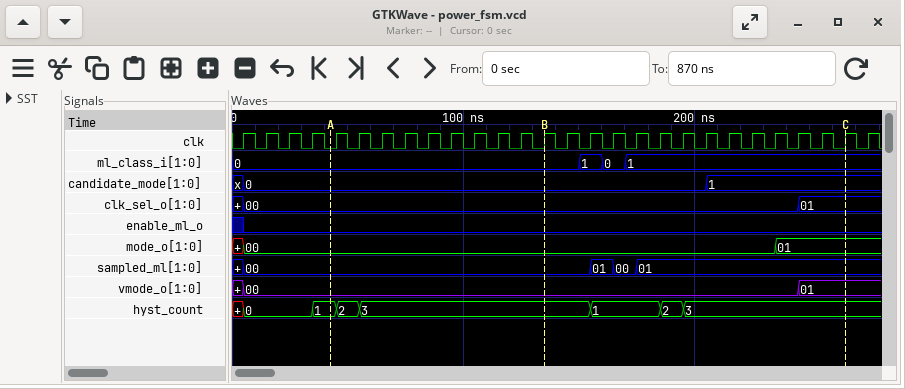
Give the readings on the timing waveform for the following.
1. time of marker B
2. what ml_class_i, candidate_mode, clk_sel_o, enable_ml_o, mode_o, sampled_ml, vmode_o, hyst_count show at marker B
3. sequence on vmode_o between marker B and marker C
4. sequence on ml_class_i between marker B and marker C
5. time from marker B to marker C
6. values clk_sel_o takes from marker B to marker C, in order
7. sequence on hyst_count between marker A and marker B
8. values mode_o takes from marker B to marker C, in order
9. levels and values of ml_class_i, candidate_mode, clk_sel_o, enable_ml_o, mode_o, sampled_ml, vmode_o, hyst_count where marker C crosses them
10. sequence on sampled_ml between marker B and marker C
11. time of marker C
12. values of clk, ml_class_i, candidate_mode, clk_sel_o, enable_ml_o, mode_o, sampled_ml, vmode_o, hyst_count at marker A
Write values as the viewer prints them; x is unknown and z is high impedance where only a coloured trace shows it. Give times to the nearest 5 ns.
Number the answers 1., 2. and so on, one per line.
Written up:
1. 135 ns
2. ml_class_i=0, candidate_mode=0, clk_sel_o=00, enable_ml_o=0, mode_o=00, sampled_ml=00, vmode_o=00, hyst_count=3
3. 00, 01
4. 0, 1, 0, 1
5. 130 ns
6. 00, 01
7. 1, 2, 3
8. 00, 01
9. ml_class_i=1, candidate_mode=1, clk_sel_o=01, enable_ml_o=0, mode_o=01, sampled_ml=01, vmode_o=01, hyst_count=3
10. 00, 01, 00, 01
11. 265 ns
12. clk=0, ml_class_i=0, candidate_mode=0, clk_sel_o=00, enable_ml_o=0, mode_o=00, sampled_ml=00, vmode_o=00, hyst_count=1
